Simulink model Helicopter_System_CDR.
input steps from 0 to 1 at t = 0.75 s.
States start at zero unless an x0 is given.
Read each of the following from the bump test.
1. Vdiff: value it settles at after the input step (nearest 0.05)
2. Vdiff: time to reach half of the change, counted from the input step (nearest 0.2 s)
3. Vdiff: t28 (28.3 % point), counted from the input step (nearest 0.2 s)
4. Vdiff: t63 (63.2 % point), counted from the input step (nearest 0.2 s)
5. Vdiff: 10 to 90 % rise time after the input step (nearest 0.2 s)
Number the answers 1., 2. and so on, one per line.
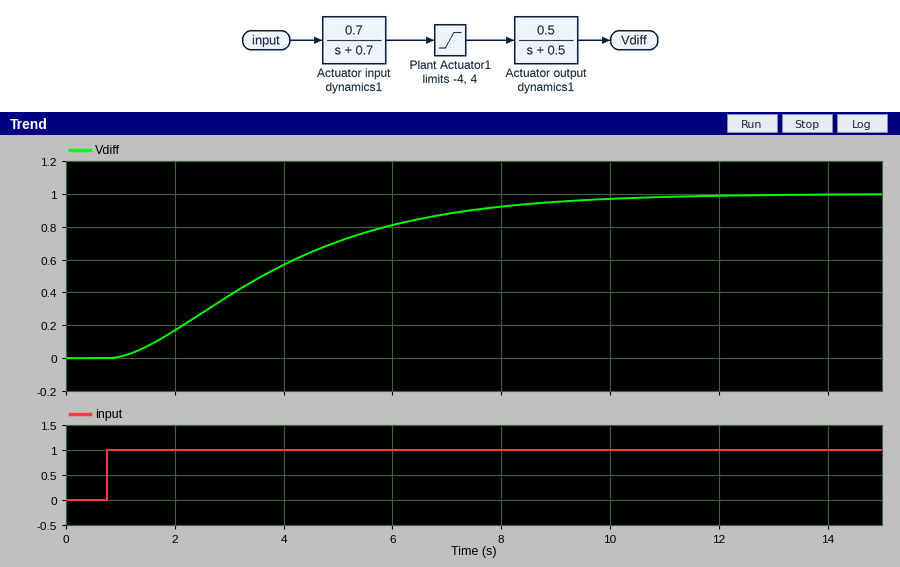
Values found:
1. 1.00
2. 2.8 s
3. 1.8 s
4. 3.6 s
5. 5.8 s
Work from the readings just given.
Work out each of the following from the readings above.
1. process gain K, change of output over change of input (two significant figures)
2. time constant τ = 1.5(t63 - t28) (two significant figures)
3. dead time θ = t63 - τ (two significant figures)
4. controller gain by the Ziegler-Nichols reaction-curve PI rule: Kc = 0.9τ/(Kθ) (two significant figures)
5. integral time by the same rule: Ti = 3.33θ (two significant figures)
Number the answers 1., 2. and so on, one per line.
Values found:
1. 1.0
2. 2.7 s
3. 0.90 s
4. 2.7
5. 3.0 s
